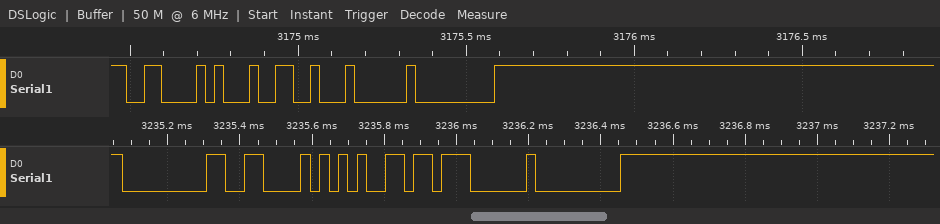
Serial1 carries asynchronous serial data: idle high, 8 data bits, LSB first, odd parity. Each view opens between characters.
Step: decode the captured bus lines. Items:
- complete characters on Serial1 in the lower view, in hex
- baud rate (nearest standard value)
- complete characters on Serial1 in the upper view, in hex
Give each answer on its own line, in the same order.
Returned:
00, 86, 65, 07, 00
38400 baud
86, 64, 04, 00
